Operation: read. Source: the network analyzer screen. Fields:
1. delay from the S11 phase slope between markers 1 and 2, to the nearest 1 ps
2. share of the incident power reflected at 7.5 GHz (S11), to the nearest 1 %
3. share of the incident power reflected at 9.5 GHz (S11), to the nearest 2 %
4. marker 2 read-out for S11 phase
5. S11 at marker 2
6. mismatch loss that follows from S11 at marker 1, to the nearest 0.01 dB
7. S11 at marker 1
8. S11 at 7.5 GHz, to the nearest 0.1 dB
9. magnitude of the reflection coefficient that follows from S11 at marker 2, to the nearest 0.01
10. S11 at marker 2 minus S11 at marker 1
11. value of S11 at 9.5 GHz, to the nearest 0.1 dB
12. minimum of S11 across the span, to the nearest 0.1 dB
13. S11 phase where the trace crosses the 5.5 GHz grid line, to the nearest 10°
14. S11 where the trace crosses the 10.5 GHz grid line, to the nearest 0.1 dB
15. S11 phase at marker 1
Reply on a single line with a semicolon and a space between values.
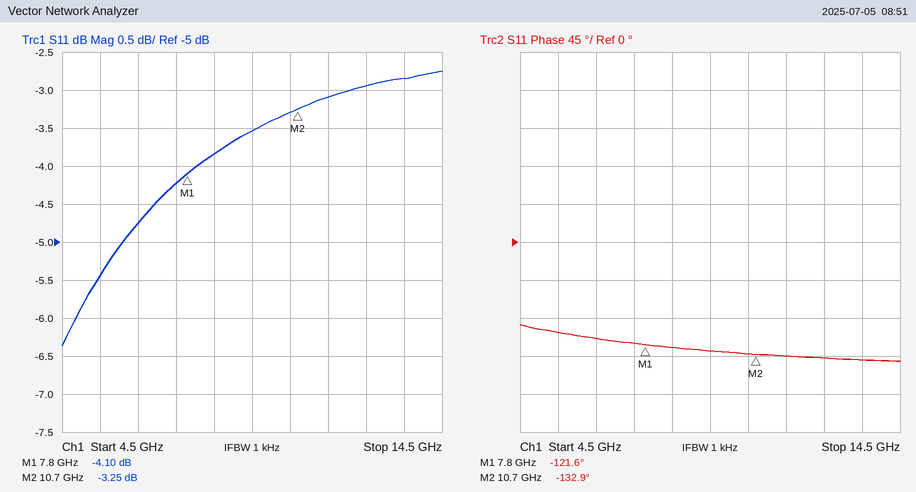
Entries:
11 ps; 38 %; 44 %; -132.9°; -3.25 dB; 2.14 dB; -4.10 dB; -4.2 dB; 0.69; 0.85 dB; -3.5 dB; -6.4 dB; -110°; -3.3 dB; -121.6°
